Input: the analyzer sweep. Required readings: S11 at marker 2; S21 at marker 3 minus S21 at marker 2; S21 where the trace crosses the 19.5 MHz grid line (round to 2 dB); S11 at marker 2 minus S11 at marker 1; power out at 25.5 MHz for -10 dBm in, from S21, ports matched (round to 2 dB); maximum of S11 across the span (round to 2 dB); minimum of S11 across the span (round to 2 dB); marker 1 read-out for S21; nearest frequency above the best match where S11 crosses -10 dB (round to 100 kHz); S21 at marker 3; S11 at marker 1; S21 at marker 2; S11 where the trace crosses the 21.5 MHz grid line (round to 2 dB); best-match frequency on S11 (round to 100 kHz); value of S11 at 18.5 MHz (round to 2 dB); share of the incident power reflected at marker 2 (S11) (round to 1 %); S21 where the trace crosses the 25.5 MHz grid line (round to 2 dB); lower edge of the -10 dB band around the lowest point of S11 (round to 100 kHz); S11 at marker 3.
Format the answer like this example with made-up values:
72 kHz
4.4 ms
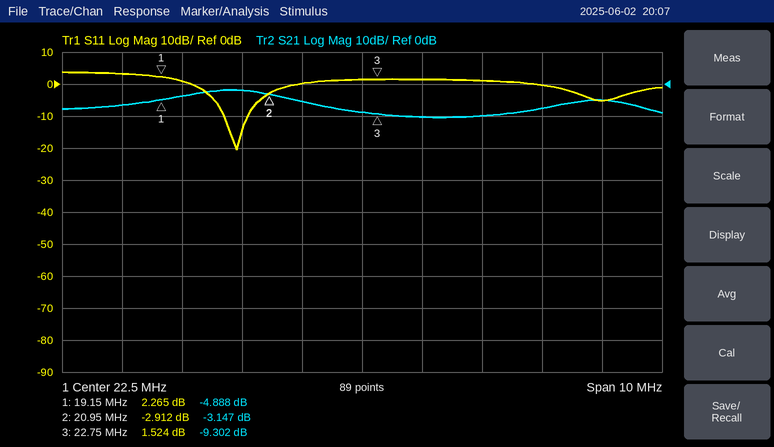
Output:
-2.912 dB
-6.155 dB
-4 dB
-5.177 dB
-18 dBm
4 dB
-20 dB
-4.888 dB
20.6 MHz
-9.302 dB
2.265 dB
-3.147 dB
0 dB
20.4 MHz
4 dB
51 %
-8 dB
20.2 MHz
1.524 dB
